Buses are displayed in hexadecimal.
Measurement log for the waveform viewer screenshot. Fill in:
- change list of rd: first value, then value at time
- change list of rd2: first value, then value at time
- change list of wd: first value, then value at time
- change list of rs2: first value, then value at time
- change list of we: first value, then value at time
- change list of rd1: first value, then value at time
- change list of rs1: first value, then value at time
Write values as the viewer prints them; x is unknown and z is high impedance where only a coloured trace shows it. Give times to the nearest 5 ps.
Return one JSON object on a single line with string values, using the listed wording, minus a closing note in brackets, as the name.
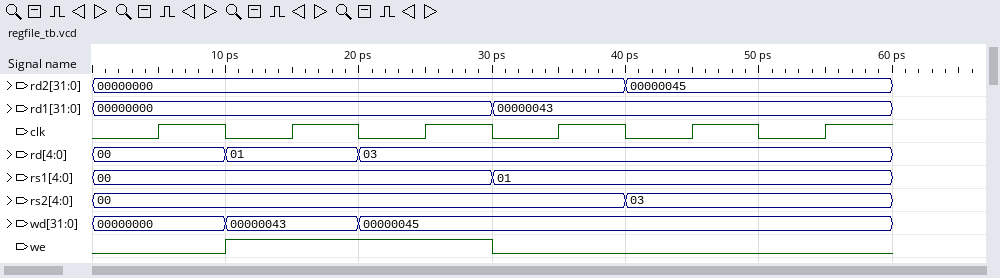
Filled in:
{"change list of rd: first value, then value at time": "00, 01 at 10 ps, 03 at 20 ps", "change list of rd2: first value, then value at time": "00000000, 00000045 at 40 ps", "change list of wd: first value, then value at time": "00000000, 00000043 at 10 ps, 00000045 at 20 ps", "change list of rs2: first value, then value at time": "00, 03 at 40 ps", "change list of we: first value, then value at time": "0, 1 at 10 ps, 0 at 30 ps", "change list of rd1: first value, then value at time": "00000000, 00000043 at 30 ps", "change list of rs1: first value, then value at time": "00, 01 at 30 ps"}
